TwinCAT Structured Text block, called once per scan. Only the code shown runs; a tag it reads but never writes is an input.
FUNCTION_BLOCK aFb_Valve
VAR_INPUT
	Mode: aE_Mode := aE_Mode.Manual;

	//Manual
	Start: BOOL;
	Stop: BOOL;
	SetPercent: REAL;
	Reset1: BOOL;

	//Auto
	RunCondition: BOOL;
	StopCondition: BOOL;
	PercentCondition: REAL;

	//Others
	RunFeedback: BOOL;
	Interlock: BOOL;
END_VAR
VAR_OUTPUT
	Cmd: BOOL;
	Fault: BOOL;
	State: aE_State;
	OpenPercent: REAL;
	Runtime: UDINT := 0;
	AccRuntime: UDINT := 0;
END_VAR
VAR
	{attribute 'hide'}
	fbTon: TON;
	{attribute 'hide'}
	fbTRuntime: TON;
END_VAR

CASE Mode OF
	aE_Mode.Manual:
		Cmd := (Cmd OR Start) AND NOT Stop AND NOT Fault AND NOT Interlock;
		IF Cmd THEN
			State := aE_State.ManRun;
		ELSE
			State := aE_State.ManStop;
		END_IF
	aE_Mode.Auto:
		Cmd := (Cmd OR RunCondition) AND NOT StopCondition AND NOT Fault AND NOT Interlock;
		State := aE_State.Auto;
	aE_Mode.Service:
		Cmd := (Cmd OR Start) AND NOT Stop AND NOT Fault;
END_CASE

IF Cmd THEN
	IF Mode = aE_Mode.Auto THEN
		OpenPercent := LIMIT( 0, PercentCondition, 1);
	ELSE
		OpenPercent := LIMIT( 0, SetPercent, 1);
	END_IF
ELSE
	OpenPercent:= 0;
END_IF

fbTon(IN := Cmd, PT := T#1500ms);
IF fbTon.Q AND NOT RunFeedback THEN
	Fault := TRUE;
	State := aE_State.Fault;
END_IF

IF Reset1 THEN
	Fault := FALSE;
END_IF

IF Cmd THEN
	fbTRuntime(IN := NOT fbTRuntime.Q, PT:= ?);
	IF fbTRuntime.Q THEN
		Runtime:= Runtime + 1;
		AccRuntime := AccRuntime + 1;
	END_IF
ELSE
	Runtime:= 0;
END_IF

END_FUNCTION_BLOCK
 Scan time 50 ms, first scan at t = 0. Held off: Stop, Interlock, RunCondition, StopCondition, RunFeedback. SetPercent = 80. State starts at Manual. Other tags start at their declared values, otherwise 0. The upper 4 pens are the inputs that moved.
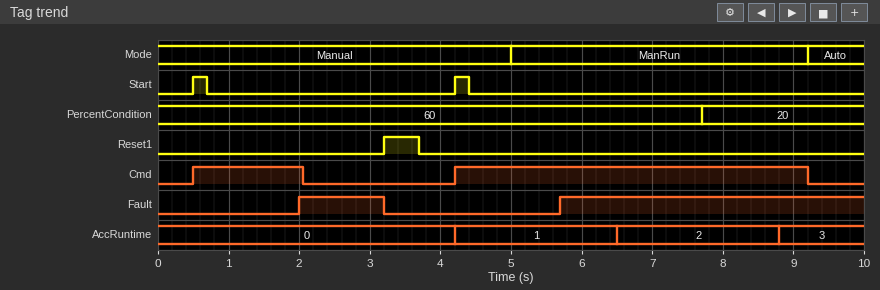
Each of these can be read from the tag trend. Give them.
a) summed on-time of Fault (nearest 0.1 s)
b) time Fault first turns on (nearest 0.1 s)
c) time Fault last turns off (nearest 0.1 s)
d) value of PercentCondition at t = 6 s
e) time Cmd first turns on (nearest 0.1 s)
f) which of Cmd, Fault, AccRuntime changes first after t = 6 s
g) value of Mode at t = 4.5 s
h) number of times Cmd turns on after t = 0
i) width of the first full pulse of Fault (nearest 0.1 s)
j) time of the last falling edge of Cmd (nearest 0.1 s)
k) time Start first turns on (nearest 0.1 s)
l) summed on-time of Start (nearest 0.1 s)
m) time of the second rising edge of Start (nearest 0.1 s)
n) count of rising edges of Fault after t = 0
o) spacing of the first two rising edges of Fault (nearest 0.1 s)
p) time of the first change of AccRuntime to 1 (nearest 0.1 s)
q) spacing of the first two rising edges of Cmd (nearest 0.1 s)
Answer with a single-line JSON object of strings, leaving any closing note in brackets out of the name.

{"summed on-time of Fault": "5.5 s", "time Fault first turns on": "2.0 s", "time Fault last turns off": "3.2 s", "value of PercentCondition at t = 6 s": "60", "time Cmd first turns on": "0.5 s", "which of Cmd, Fault, AccRuntime changes first after t = 6 s": "AccRuntime", "value of Mode at t = 4.5 s": "Manual", "number of times Cmd turns on after t = 0": "2", "width of the first full pulse of Fault": "1.2 s", "time of the last falling edge of Cmd": "9.2 s", "time Start first turns on": "0.5 s", "summed on-time of Start": "0.4 s", "time of the second rising edge of Start": "4.2 s", "count of rising edges of Fault after t = 0": "2", "spacing of the first two rising edges of Fault": "3.7 s", "time of the first change of AccRuntime to 1": "4.2 s", "spacing of the first two rising edges of Cmd": "3.7 s"}
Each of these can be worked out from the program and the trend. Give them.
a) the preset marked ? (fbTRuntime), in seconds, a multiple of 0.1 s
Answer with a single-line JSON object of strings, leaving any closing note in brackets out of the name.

{"the preset marked ? (fbTRuntime), in seconds, a multiple of 0.1 s": "2.2 s"}
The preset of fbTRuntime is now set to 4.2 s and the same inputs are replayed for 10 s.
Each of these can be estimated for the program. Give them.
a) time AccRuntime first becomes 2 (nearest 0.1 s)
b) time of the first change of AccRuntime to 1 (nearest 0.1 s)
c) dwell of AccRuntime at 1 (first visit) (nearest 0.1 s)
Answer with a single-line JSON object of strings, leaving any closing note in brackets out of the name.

{"time AccRuntime first becomes 2": "9.0 s", "time of the first change of AccRuntime to 1": "4.7 s", "dwell of AccRuntime at 1 (first visit)": "4.3 s"}
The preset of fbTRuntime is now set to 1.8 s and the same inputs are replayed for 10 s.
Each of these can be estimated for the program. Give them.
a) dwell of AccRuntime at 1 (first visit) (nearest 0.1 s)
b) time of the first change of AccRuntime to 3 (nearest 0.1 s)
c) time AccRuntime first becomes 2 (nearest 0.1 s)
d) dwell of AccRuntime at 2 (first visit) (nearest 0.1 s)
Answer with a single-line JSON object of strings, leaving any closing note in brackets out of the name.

{"dwell of AccRuntime at 1 (first visit)": "1.9 s", "time of the first change of AccRuntime to 3": "8.0 s", "time AccRuntime first becomes 2": "6.1 s", "dwell of AccRuntime at 2 (first visit)": "1.9 s"}
